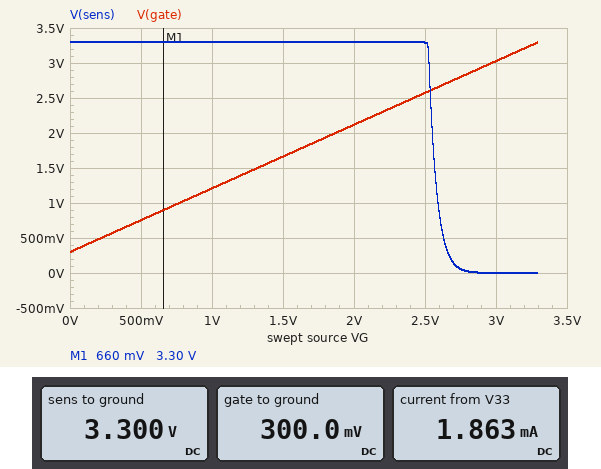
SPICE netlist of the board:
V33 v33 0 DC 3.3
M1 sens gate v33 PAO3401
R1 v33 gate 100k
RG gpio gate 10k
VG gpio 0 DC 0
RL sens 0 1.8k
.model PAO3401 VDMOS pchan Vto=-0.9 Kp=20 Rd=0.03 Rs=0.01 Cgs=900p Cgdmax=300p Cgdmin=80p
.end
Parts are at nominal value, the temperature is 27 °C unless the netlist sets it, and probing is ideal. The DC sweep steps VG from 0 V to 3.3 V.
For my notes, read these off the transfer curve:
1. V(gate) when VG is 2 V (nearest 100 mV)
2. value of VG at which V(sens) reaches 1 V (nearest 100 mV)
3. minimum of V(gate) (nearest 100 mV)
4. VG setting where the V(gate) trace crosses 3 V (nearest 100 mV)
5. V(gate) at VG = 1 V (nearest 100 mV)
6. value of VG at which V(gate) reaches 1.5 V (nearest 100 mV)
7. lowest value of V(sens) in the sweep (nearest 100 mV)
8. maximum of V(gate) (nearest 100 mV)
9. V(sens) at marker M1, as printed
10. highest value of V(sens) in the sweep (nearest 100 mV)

2.1 V
2.6 V
300 mV
3.0 V
1.2 V
1.3 V
0 V
3.3 V
3.30 V
3.3 V
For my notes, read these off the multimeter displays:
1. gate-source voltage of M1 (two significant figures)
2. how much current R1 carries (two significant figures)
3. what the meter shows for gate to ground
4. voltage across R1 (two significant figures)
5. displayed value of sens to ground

-3.0 V
30 µA
300.0 mV
3.0 V
3.300 V
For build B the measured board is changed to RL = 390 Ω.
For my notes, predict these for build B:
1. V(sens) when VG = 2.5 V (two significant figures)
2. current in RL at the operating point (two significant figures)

1.0 V
8.5 mA
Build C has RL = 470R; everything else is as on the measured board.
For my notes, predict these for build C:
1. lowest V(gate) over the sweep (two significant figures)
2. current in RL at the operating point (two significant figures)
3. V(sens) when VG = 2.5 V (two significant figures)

300 mV
7.0 mA
1.3 V
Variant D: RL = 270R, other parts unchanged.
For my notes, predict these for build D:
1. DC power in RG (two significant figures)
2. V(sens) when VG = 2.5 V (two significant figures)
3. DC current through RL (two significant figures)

9.0 µW
720 mV
12 mA
